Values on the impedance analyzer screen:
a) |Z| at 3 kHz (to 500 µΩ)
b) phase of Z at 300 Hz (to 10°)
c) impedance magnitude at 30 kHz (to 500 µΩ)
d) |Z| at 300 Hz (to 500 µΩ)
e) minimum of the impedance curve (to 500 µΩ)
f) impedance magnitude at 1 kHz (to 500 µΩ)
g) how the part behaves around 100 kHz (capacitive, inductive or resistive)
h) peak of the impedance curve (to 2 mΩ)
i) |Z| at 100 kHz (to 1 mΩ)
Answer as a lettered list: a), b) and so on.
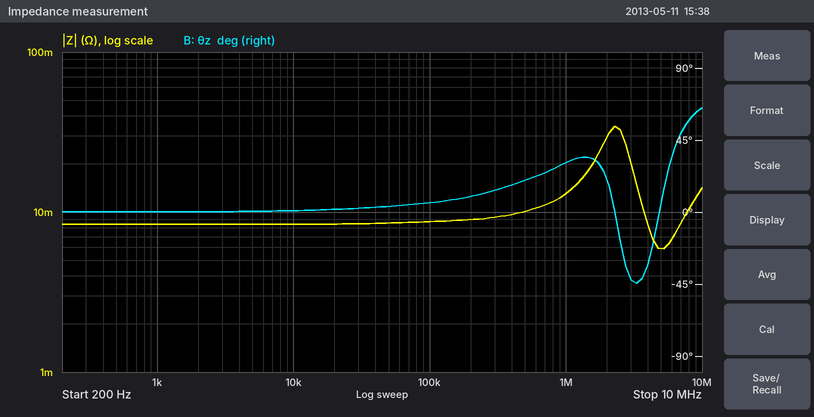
a) 8.5 mΩ
b) 0°
c) 8.5 mΩ
d) 8.5 mΩ
e) 6.0 mΩ
f) 8.5 mΩ
g) resistive
h) 34 mΩ
i) 9 mΩ
